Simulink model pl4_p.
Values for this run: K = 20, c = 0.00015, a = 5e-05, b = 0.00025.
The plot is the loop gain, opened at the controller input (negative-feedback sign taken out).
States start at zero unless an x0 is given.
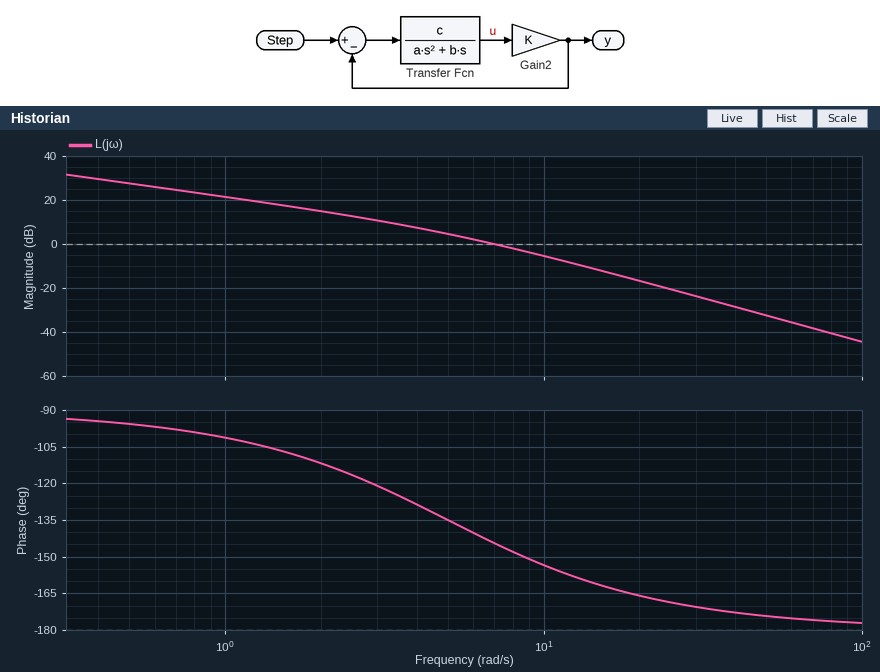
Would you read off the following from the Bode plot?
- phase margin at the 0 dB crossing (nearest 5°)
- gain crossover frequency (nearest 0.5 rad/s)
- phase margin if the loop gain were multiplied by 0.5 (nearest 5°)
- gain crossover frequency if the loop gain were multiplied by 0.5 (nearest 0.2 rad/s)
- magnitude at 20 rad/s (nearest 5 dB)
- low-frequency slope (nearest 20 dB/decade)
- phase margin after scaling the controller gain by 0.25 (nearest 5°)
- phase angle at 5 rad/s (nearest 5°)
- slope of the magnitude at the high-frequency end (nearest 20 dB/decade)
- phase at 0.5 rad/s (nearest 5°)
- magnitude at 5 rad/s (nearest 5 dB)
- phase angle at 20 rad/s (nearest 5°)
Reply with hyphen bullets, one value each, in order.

- 35°
- 7.0 rad/s
- 50°
- 4.4 rad/s
- -15 dB
- -20 dB/decade
- 60°
- -135°
- -40 dB/decade
- -95°
- 5 dB
- -165°
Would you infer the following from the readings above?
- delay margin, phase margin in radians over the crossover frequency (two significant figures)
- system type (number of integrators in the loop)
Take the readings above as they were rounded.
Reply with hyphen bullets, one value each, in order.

- 0.087 s
- 1
